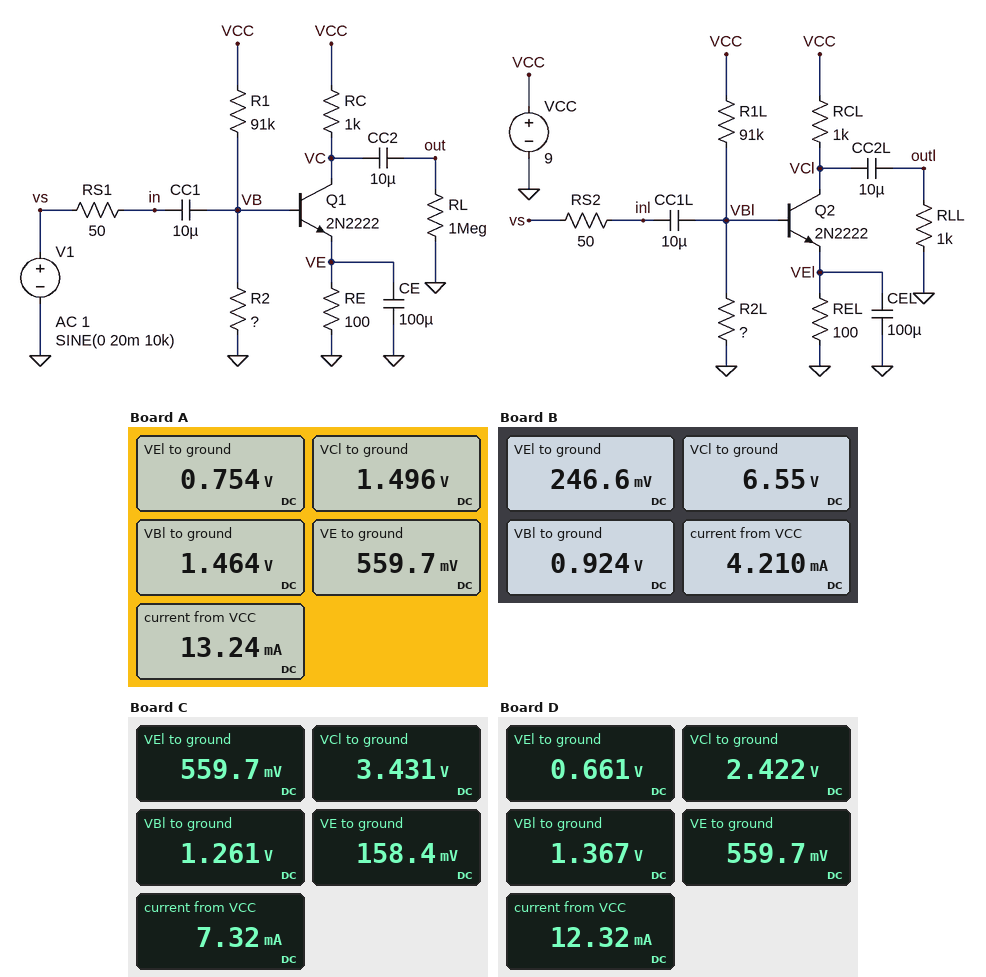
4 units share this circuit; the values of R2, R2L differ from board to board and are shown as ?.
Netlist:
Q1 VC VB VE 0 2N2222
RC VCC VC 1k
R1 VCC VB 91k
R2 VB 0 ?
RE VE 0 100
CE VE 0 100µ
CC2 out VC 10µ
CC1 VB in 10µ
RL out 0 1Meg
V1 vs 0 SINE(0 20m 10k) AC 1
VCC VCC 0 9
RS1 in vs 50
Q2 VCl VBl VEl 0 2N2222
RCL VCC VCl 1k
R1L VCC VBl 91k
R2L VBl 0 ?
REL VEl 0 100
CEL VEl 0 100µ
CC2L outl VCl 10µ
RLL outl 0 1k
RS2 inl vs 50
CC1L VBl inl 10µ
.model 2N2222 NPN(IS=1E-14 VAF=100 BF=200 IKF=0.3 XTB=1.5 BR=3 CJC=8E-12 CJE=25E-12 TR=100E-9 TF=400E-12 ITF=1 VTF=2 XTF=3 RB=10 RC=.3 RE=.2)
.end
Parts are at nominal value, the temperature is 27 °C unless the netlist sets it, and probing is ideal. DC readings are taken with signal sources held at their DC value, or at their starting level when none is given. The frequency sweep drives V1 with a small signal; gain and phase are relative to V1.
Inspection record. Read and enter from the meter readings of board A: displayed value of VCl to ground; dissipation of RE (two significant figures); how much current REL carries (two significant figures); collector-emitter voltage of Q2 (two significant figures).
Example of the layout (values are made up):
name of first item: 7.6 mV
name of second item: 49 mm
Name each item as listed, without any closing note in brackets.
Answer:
displayed value of VCl to ground: 1.496 V
dissipation of RE: 3.1 mW
how much current REL carries: 7.5 mA
collector-emitter voltage of Q2: 740 mV
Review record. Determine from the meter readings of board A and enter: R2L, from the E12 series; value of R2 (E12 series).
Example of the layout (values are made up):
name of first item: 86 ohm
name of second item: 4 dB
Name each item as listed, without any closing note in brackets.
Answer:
R2L, from the E12 series: 33 kΩ
value of R2: 22 kΩ
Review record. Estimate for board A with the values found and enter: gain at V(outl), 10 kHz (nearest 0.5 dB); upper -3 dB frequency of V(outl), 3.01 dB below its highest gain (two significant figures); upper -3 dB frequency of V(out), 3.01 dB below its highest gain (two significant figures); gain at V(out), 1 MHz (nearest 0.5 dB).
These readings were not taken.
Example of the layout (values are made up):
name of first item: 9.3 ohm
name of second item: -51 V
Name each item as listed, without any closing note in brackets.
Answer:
gain at V(outl), 10 kHz: 41.5 dB
upper -3 dB frequency of V(outl), 3.01 dB below its highest gain: 2.3 MHz
upper -3 dB frequency of V(out), 3.01 dB below its highest gain: 2.4 MHz
gain at V(out), 1 MHz: 44.5 dB
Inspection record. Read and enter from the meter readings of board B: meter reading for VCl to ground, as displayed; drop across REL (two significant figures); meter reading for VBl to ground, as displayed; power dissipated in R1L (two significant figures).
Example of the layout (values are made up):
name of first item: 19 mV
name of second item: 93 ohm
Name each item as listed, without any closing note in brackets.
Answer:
meter reading for VCl to ground, as displayed: 6.55 V
drop across REL: 250 mV
meter reading for VBl to ground, as displayed: 0.924 V
power dissipated in R1L: 720 µW
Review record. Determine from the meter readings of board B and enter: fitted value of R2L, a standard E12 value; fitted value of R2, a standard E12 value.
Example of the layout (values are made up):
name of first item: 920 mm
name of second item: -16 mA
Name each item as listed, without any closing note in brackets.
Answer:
fitted value of R2L, a standard E12 value: 12 kΩ
fitted value of R2, a standard E12 value: 10 kΩ
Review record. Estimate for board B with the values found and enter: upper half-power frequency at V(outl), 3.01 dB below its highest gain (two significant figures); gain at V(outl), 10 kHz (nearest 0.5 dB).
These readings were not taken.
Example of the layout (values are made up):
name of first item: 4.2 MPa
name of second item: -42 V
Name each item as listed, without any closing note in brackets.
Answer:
upper half-power frequency at V(outl), 3.01 dB below its highest gain: 9.6 MHz
gain at V(outl), 10 kHz: 33.0 dB
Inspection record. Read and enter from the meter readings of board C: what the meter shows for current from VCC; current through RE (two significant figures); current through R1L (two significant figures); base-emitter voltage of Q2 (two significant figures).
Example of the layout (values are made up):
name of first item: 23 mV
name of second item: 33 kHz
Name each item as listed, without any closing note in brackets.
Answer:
what the meter shows for current from VCC: 7.32 mA
current through RE: 1.6 mA
current through R1L: 85 µA
base-emitter voltage of Q2: 700 mV
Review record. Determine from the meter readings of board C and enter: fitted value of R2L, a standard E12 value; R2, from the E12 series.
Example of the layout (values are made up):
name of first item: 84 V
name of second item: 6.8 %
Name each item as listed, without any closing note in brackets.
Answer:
fitted value of R2L, a standard E12 value: 22 kΩ
R2, from the E12 series: 10 kΩ
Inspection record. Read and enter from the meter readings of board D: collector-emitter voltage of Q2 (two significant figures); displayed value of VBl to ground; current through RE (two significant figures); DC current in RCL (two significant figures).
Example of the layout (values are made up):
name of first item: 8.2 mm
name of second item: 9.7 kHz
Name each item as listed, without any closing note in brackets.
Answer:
collector-emitter voltage of Q2: 1.8 V
displayed value of VBl to ground: 1.367 V
current through RE: 5.6 mA
DC current in RCL: 6.6 mA
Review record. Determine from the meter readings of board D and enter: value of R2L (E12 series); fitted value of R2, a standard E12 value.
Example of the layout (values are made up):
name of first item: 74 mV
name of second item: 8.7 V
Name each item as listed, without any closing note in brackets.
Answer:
value of R2L: 27 kΩ
fitted value of R2, a standard E12 value: 22 kΩ
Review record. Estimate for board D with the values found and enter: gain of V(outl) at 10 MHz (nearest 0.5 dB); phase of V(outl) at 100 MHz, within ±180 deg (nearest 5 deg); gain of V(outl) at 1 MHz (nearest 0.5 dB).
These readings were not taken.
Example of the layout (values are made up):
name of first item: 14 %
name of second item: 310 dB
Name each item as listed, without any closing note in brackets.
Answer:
gain of V(outl) at 10 MHz: 30.5 dB
phase of V(outl) at 100 MHz, within ±180 deg: 75 deg
gain of V(outl) at 1 MHz: 40.0 dB
